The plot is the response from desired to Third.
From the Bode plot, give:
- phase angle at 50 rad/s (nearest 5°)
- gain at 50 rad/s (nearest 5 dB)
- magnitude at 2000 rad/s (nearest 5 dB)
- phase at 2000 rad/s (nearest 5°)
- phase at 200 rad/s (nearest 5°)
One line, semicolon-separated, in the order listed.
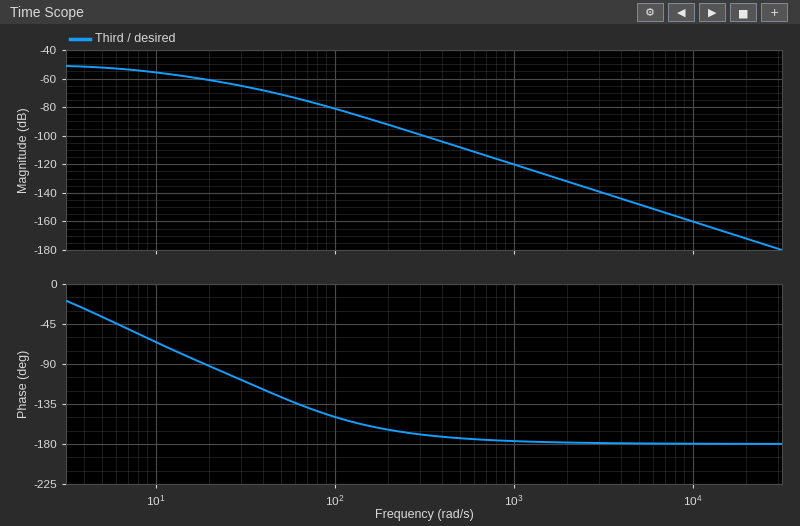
-125°; -70 dB; -130 dB; -180°; -165°
